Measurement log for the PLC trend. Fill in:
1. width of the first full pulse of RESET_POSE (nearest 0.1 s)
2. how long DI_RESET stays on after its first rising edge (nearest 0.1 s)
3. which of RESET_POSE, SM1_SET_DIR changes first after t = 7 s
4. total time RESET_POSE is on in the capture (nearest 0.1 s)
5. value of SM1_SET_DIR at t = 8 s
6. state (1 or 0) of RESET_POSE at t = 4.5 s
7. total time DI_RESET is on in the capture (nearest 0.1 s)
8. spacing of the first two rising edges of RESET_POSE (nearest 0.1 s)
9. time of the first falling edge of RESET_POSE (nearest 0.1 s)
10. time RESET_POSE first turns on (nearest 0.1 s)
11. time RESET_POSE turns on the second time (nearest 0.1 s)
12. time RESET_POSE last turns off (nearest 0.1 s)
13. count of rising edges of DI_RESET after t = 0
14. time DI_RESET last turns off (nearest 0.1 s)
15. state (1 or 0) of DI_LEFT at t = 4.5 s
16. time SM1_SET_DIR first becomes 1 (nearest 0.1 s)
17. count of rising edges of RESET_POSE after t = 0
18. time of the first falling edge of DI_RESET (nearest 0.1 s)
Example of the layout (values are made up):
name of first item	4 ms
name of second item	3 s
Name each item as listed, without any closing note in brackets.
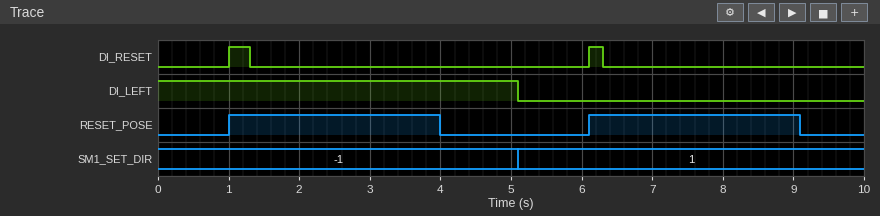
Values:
width of the first full pulse of RESET_POSE	3.0 s
how long DI_RESET stays on after its first rising edge	0.3 s
which of RESET_POSE, SM1_SET_DIR changes first after t = 7 s	RESET_POSE
total time RESET_POSE is on in the capture	6.0 s
value of SM1_SET_DIR at t = 8 s	1
state (1 or 0) of RESET_POSE at t = 4.5 s	0
total time DI_RESET is on in the capture	0.5 s
spacing of the first two rising edges of RESET_POSE	5.1 s
time of the first falling edge of RESET_POSE	4.0 s
time RESET_POSE first turns on	1.0 s
time RESET_POSE turns on the second time	6.1 s
time RESET_POSE last turns off	9.1 s
count of rising edges of DI_RESET after t = 0	2
time DI_RESET last turns off	6.3 s
state (1 or 0) of DI_LEFT at t = 4.5 s	1
time SM1_SET_DIR first becomes 1	5.1 s
count of rising edges of RESET_POSE after t = 0	2
time of the first falling edge of DI_RESET	1.3 s
